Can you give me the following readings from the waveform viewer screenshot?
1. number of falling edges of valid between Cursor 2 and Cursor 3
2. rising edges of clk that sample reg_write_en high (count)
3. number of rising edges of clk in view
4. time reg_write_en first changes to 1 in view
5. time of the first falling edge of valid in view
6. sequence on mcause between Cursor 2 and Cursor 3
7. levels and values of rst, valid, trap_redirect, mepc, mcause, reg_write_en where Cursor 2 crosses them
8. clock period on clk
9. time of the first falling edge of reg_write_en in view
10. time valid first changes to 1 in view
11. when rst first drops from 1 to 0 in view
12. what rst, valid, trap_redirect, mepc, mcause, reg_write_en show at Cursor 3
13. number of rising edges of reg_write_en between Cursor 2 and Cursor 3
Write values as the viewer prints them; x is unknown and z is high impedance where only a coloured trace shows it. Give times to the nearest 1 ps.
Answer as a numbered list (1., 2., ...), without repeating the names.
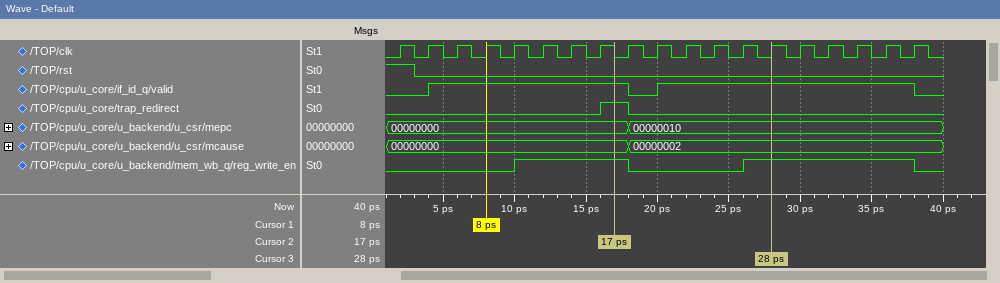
1. 1
2. 10
3. 19
4. 10 ps
5. 18 ps
6. 00000000, 00000002
7. rst=0, valid=1, trap_redirect=1, mepc=00000000, mcause=00000000, reg_write_en=1
8. 2 ps
9. 18 ps
10. 4 ps
11. 3 ps
12. rst=0, valid=1, trap_redirect=0, mepc=00000010, mcause=00000002, reg_write_en=1
13. 1
